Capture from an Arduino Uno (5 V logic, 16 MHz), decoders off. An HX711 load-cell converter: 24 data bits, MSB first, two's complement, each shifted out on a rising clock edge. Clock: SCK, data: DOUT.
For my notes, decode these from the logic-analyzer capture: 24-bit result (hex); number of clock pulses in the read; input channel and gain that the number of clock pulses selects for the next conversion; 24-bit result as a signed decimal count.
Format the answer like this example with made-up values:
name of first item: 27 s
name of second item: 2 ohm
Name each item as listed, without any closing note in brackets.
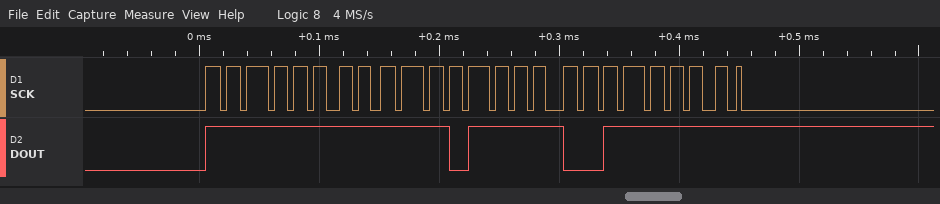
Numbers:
24-bit result: 0xFFEF3F
number of clock pulses in the read: 25
input channel and gain that the number of clock pulses selects for the next conversion: channel A, gain 128
24-bit result as a signed decimal count: -4289
